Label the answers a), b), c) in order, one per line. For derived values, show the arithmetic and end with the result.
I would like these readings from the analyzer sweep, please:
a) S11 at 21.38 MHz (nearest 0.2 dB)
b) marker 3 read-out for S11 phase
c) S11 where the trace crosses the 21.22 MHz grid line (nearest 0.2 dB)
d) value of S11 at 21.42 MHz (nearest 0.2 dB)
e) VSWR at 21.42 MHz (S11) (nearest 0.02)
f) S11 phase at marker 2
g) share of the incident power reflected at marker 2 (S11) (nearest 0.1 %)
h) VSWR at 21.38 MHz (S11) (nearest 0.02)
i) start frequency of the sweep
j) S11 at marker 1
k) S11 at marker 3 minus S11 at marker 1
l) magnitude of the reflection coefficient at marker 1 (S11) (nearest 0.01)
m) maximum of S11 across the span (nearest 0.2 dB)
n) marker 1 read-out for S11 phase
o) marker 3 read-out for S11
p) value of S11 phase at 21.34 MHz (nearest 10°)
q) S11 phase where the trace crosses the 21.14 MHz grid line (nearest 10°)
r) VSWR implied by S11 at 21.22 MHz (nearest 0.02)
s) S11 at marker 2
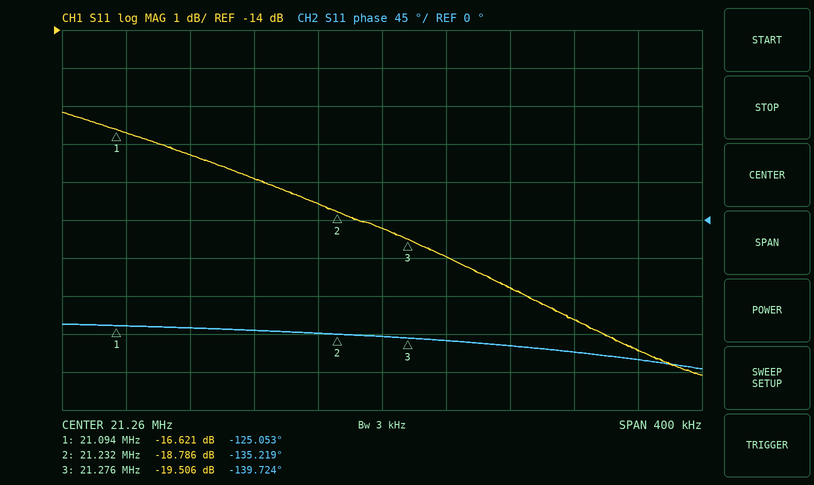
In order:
a) -21.6 dB
b) -139.724°
c) -18.6 dB
d) -22.4 dB
e) |Γ| = 10^(-22.4/20) = 0.0759; VSWR = (1 + 0.0759)/(1 − 0.0759) ≈ 1.16
f) -135.219°
g) 10^(-18.786/10) ≈ 1.3 %
h) |Γ| = 10^(-21.6/20) = 0.0832; VSWR = (1 + 0.0832)/(1 − 0.0832) ≈ 1.18
i) 21.06 MHz
j) -16.621 dB
k) -19.506 − (-16.621) = -2.885 dB
l) 10^(-16.621/20) ≈ 0.15
m) -16.2 dB
n) -125.053°
o) -19.506 dB
p) -150°
q) -130°
r) |Γ| = 10^(-18.6/20) = 0.1175; VSWR = (1 + 0.1175)/(1 − 0.1175) ≈ 1.27, so 1.26 to the nearest 0.02
s) -18.786 dB
